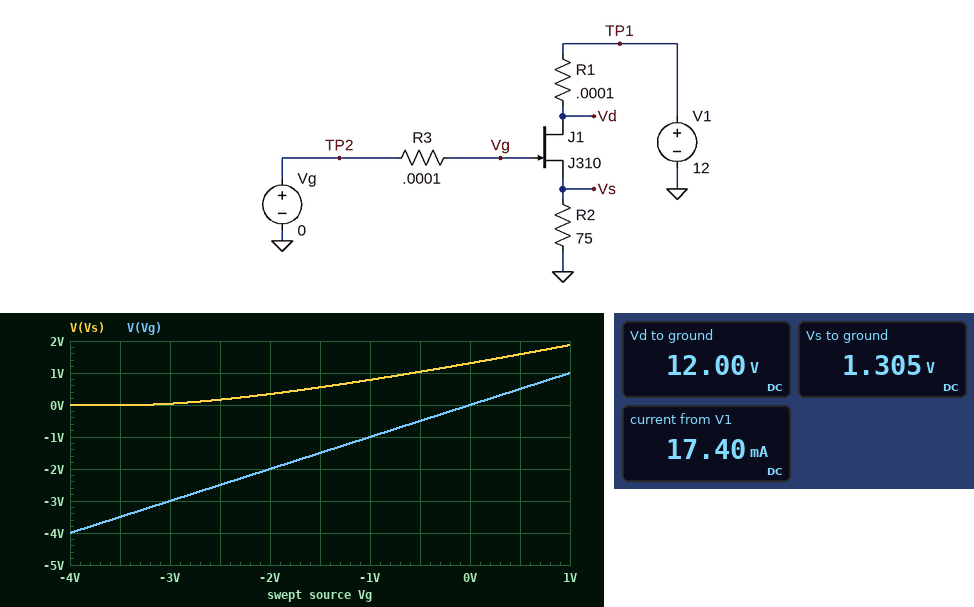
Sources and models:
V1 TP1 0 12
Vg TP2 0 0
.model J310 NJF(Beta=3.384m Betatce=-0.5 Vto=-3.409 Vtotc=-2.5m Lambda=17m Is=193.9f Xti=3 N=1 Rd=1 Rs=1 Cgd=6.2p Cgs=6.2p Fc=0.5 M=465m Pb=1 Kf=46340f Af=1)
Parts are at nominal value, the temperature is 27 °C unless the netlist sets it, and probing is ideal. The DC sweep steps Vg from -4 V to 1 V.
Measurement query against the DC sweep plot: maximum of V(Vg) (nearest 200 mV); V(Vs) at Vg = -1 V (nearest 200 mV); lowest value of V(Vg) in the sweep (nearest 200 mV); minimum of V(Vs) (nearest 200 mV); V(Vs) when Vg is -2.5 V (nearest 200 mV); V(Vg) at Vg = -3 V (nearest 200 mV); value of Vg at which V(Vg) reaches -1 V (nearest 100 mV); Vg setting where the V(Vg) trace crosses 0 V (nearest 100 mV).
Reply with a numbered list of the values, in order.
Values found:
1. 1.0 V
2. 800 mV
3. -4.0 V
4. 0 V
5. 200 mV
6. -3.0 V
7. -1.0 V
8. 0 V
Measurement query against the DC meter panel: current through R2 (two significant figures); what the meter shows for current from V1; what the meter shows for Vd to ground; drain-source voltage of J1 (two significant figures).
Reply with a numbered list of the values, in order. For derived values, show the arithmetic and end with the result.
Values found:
1. (1.305 V) / 75 Ω = 17 mA
2. 17.40 mA
3. 12.00 V
4. 12 V - 1.305 V = 11 V
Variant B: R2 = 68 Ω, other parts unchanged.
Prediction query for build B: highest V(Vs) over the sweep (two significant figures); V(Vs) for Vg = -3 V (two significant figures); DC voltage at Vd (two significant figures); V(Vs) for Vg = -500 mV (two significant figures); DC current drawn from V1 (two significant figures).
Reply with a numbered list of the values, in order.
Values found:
1. 1.8 V
2. 38 mV
3. 12 V
4. 990 mV
5. 18 mA
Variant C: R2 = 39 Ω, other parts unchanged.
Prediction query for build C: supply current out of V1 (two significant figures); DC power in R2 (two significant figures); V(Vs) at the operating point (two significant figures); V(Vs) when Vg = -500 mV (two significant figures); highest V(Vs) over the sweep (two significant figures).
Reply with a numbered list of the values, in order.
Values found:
1. 24 mA
2. 23 mW
3. 940 mV
4. 730 mV
5. 1.4 V
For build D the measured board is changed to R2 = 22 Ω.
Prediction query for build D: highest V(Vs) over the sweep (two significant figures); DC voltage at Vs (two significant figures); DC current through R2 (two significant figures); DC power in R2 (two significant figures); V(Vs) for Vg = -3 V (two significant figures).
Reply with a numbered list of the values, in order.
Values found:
1. 1.0 V
2. 660 mV
3. 30 mA
4. 20 mW
5. 14 mV
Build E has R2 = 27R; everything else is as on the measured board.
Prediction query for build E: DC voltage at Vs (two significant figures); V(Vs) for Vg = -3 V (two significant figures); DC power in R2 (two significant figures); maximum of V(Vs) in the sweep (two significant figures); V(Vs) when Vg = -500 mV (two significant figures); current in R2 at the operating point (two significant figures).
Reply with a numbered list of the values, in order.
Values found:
1. 750 mV
2. 17 mV
3. 21 mW
4. 1.1 V
5. 580 mV
6. 28 mA
